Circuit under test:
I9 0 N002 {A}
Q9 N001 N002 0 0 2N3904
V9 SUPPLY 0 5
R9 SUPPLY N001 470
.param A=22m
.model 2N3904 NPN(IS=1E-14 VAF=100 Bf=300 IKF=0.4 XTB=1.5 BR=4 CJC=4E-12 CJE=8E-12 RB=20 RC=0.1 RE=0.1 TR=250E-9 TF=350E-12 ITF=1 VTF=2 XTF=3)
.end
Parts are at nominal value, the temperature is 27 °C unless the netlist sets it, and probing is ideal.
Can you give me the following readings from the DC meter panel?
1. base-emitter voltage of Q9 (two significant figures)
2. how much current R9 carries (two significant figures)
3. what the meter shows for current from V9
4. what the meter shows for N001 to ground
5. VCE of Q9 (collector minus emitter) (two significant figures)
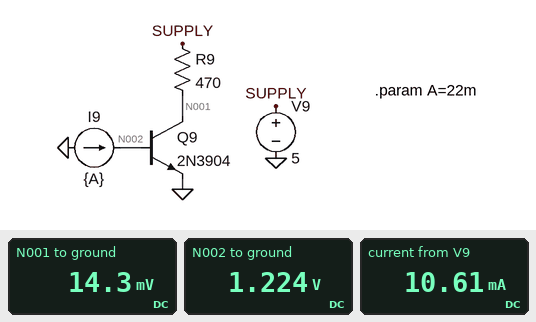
1.2 V
11 mA
10.61 mA
14.3 mV
14 mV
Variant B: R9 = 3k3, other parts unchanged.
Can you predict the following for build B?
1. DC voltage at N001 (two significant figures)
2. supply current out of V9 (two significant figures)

9.9 mV
1.5 mA
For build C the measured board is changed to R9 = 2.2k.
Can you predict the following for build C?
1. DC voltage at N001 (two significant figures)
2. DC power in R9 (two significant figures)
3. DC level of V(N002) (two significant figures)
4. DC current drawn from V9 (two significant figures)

10 mV
11 mW
1.2 V
2.3 mA
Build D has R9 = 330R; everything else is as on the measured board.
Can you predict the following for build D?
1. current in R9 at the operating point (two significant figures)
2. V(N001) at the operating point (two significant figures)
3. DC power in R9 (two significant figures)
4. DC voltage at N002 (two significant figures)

15 mA
16 mV
75 mW
1.2 V
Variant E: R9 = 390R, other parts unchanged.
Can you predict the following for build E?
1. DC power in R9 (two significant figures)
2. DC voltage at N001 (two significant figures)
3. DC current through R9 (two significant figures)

64 mW
15 mV
13 mA
